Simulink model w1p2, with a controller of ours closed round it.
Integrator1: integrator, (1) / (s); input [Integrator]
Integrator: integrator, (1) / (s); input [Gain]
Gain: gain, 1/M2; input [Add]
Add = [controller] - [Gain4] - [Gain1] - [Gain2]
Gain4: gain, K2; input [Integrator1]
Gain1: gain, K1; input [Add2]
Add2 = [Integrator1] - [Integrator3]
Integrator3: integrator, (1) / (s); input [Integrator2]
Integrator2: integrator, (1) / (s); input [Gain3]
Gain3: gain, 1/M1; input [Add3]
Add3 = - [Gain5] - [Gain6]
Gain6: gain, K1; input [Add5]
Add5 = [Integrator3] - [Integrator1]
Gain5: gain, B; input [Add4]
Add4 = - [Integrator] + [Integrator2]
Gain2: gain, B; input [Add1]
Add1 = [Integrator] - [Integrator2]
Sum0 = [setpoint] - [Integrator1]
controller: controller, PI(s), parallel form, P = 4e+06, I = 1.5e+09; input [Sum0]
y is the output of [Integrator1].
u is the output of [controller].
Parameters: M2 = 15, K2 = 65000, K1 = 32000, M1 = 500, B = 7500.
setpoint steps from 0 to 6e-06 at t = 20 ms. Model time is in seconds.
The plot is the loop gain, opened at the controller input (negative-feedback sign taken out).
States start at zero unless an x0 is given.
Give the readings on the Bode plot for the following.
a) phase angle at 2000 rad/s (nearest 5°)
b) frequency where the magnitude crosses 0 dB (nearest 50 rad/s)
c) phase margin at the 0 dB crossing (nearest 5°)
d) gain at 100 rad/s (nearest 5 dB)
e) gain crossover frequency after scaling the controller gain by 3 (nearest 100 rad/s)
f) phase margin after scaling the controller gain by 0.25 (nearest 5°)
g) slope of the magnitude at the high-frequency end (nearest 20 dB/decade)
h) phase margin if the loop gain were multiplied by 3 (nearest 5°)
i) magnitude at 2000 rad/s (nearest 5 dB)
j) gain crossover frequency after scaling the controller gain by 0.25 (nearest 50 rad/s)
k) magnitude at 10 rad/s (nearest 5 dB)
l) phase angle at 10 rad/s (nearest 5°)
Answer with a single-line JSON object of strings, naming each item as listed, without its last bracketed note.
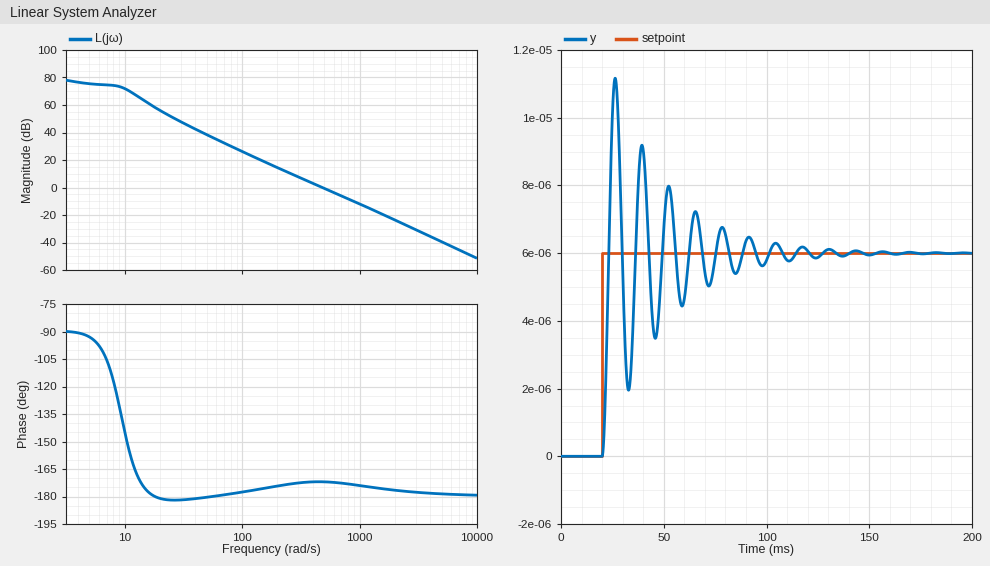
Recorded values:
{"phase angle at 2000 rad/s": "-175°", "frequency where the magnitude crosses 0 dB": "500 rad/s", "phase margin at the 0 dB crossing": "10°", "gain at 100 rad/s": "25 dB", "gain crossover frequency after scaling the controller gain by 3": "900 rad/s", "phase margin after scaling the controller gain by 0.25": "5°", "slope of the magnitude at the high-frequency end": "-40 dB/decade", "phase margin if the loop gain were multiplied by 3": "5°", "magnitude at 2000 rad/s": "-25 dB", "gain crossover frequency after scaling the controller gain by 0.25": "250 rad/s", "magnitude at 10 rad/s": "70 dB", "phase angle at 10 rad/s": "-145°"}
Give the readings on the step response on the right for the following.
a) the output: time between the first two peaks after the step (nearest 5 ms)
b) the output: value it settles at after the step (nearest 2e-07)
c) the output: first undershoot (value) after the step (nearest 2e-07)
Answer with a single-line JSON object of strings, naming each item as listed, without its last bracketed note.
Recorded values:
{"the output: time between the first two peaks after the step": "15 ms", "the output: value it settles at after the step": "0.0000060", "the output: first undershoot (value) after the step": "0.0000020"}
